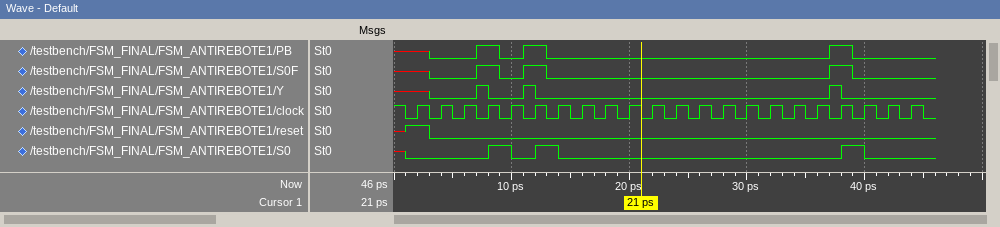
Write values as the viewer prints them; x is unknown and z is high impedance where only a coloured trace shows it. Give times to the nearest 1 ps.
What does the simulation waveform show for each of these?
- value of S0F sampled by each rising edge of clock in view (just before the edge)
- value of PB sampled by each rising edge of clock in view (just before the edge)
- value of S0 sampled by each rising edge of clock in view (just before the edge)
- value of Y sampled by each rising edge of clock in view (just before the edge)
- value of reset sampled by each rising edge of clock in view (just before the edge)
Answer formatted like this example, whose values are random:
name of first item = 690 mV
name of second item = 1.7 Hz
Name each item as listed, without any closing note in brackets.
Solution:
value of S0F sampled by each rising edge of clock in view = x 0 0 1 0 1 0 0 0 0 0 0 0 0 0 0 0 0 1 0 0 0
value of PB sampled by each rising edge of clock in view = x 0 0 1 0 1 0 0 0 0 0 0 0 0 0 0 0 0 1 0 0 0
value of S0 sampled by each rising edge of clock in view = 0 0 0 0 1 0 1 0 0 0 0 0 0 0 0 0 0 0 0 1 0 0
value of Y sampled by each rising edge of clock in view = x 0 0 1 0 1 0 0 0 0 0 0 0 0 0 0 0 0 1 0 0 0
value of reset sampled by each rising edge of clock in view = 1 0 0 0 0 0 0 0 0 0 0 0 0 0 0 0 0 0 0 0 0 0
